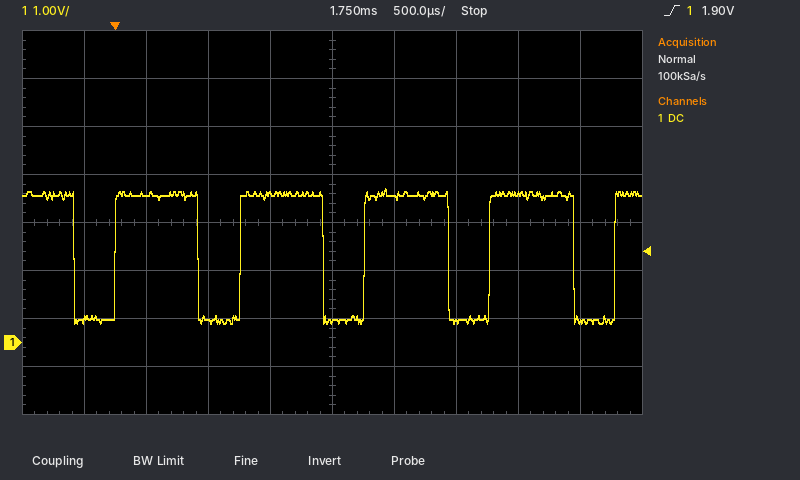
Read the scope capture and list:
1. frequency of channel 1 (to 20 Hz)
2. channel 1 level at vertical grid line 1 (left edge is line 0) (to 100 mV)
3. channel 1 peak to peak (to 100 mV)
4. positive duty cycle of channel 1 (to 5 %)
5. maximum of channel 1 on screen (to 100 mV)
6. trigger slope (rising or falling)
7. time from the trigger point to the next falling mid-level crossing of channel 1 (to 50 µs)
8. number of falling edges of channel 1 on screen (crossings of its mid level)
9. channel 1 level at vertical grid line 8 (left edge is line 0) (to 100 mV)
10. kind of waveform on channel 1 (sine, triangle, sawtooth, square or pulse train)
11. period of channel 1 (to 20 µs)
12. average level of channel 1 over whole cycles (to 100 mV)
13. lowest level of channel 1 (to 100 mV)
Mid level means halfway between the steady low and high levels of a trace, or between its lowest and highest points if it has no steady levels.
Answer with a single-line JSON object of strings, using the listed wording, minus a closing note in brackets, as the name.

{"frequency of channel 1": "1.00 kHz", "channel 1 level at vertical grid line 1 (left edge is line 0)": "500 mV", "channel 1 peak to peak": "2.8 V", "positive duty cycle of channel 1": "65 %", "maximum of channel 1 on screen": "3.2 V", "trigger slope": "rising", "time from the trigger point to the next falling mid-level crossing of channel 1": "650 µs", "number of falling edges of channel 1 on screen": "5", "channel 1 level at vertical grid line 8 (left edge is line 0)": "3.1 V", "kind of waveform on channel 1": "pulse train", "period of channel 1": "1.00 ms", "average level of channel 1 over whole cycles": "2.2 V", "lowest level of channel 1": "400 mV"}
